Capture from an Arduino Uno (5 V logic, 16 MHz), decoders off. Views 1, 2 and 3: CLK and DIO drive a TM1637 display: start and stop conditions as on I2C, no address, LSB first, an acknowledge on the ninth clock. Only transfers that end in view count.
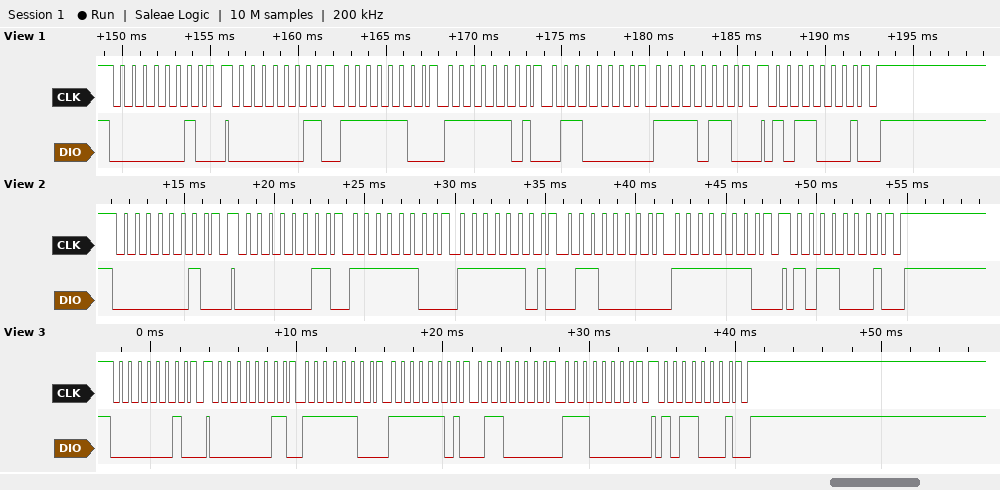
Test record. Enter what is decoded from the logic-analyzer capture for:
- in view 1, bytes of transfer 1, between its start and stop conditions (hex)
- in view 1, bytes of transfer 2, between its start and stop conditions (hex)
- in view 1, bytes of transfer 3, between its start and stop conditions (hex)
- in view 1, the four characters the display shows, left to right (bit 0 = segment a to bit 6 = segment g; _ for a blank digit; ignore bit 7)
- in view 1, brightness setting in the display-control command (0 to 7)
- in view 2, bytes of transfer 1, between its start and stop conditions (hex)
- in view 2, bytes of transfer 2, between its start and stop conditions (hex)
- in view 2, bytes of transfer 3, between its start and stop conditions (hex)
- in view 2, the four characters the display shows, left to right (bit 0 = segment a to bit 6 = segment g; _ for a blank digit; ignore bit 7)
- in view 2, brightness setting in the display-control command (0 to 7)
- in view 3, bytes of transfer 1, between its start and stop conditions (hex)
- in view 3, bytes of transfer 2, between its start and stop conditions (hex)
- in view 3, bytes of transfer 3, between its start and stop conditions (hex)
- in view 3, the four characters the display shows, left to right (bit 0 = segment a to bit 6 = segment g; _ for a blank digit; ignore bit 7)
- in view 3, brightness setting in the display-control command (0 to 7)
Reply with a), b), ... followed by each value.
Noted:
a) 40
b) C0 3F BF 06 6F
c) 8D
d) 0019
e) 5
f) 40
g) C0 3F BF 06 7F
h) 8D
i) 0018
j) 5
k) 40
l) C0 3F BF 06 07
m) 8D
n) 0017
o) 5
